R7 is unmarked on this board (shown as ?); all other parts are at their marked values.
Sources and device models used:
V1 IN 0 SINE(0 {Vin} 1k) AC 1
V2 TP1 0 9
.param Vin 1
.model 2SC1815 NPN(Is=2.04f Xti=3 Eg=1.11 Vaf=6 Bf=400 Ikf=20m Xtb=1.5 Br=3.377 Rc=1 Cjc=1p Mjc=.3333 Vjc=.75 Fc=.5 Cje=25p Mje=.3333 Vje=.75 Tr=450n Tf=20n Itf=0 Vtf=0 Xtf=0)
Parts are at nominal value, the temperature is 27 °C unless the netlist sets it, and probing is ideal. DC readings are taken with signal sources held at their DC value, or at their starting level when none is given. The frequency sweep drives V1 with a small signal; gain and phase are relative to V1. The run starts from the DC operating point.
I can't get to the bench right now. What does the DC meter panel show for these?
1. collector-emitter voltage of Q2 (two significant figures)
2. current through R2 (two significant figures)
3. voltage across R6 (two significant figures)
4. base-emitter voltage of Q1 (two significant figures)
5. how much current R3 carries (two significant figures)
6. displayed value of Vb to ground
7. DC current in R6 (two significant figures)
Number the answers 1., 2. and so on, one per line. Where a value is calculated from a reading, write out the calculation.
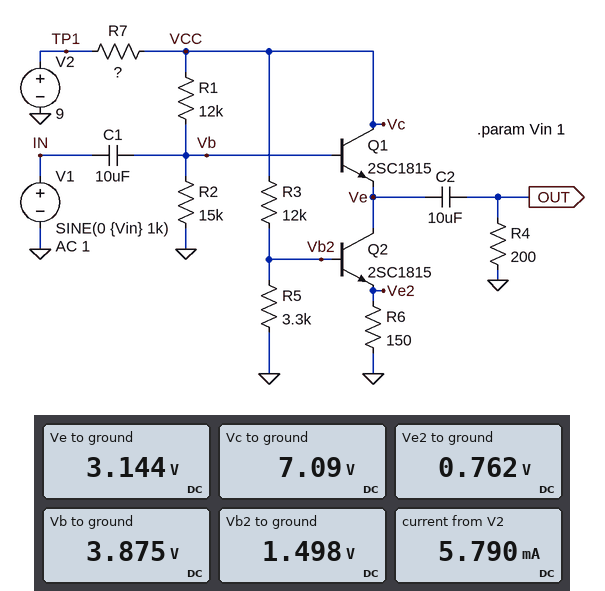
1. 3.144 V - 762 mV = 2.4 V
2. (3.875 V) / 15 kΩ = 260 µA
3. 762 mV = 760 mV
4. 3.875 V - 3.144 V = 730 mV
5. (7.09 V - 1.498 V) / 12 kΩ = 470 µA
6. 3.875 V
7. (762 mV) / 150 Ω = 5.1 mA
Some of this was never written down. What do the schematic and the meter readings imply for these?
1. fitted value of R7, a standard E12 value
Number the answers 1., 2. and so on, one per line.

1. 330 Ω
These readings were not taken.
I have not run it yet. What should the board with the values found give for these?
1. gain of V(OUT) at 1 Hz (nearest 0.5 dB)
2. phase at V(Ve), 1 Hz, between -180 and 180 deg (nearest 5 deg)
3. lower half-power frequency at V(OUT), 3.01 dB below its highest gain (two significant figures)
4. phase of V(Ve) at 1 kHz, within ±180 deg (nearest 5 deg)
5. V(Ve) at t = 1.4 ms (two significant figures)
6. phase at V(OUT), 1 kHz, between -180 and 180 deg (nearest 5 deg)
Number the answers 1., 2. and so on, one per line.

1. -46.5 dB
2. 65 deg
3. 79 Hz
4. 0 deg
5. 3.7 V
6. 5 deg
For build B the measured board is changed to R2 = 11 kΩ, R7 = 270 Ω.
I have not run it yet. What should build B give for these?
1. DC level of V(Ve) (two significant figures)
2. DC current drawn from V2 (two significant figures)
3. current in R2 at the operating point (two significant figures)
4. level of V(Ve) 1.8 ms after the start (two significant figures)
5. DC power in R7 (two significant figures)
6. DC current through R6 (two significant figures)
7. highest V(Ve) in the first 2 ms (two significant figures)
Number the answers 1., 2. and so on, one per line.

1. 2.7 V
2. 6.2 mA
3. 310 µA
4. 1.8 V
5. 10 mW
6. 5.4 mA
7. 3.7 V
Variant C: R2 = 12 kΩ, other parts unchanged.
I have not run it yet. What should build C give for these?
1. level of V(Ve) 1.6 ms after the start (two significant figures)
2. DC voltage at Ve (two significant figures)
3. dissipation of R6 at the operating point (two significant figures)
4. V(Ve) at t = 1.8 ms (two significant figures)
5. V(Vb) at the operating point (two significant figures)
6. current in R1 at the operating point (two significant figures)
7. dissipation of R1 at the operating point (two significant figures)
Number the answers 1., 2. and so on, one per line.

1. 2.2 V
2. 2.8 V
3. 3.8 mW
4. 1.8 V
5. 3.5 V
6. 300 µA
7. 1.1 mW
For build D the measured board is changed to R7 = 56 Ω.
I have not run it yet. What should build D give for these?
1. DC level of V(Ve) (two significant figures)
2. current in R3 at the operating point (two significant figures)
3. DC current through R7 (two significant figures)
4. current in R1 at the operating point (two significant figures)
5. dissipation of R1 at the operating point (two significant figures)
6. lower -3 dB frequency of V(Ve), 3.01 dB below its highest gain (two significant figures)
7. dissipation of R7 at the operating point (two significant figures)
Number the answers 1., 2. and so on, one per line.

1. 3.9 V
2. 560 µA
3. 7.9 mA
4. 320 µA
5. 1.3 mW
6. 2.4 Hz
7. 3.5 mW
